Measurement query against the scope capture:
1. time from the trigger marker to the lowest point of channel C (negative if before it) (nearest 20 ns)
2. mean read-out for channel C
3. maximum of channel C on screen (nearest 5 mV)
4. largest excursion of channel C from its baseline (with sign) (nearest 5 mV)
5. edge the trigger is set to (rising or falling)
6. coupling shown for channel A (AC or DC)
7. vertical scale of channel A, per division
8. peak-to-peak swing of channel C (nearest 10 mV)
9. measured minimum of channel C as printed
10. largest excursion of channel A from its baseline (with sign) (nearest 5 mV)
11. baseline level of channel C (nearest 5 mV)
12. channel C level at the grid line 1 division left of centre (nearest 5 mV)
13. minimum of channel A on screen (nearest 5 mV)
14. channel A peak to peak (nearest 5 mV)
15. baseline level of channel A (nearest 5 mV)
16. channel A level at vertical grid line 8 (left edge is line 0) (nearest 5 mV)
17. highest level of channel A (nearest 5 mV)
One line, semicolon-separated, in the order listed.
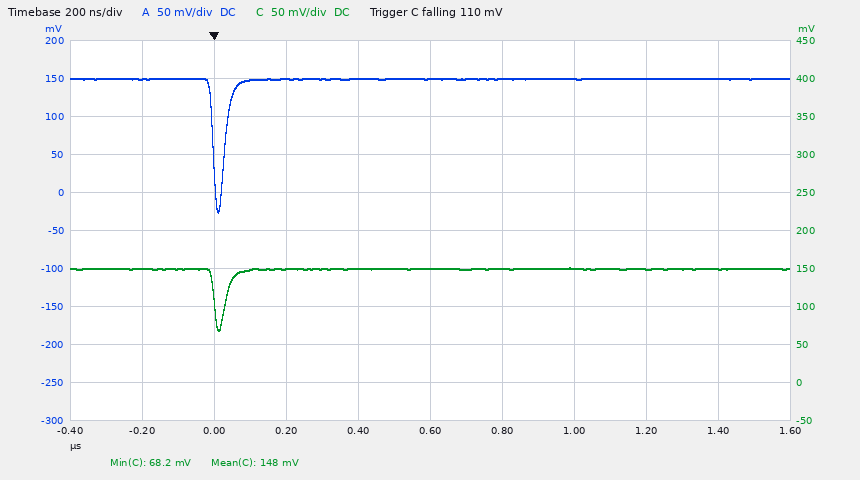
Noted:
+20 ns; 148 mV; 150 mV; -80 mV; falling; DC; 50 mV; 80 mV; 68.2 mV; -175 mV; 150 mV; 150 mV; -25 mV; 175 mV; 150 mV; 150 mV; 150 mV
